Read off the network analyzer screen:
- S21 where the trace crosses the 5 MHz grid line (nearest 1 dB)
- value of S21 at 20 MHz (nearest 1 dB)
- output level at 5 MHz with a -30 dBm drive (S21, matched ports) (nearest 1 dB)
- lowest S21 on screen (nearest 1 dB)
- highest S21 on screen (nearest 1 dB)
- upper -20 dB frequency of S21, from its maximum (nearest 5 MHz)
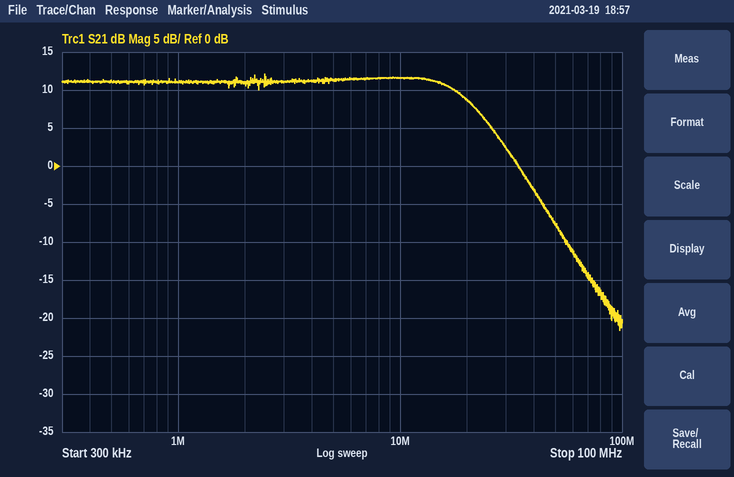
11 dB
9 dB
-19 dBm
-22 dB
12 dB
50 MHz
